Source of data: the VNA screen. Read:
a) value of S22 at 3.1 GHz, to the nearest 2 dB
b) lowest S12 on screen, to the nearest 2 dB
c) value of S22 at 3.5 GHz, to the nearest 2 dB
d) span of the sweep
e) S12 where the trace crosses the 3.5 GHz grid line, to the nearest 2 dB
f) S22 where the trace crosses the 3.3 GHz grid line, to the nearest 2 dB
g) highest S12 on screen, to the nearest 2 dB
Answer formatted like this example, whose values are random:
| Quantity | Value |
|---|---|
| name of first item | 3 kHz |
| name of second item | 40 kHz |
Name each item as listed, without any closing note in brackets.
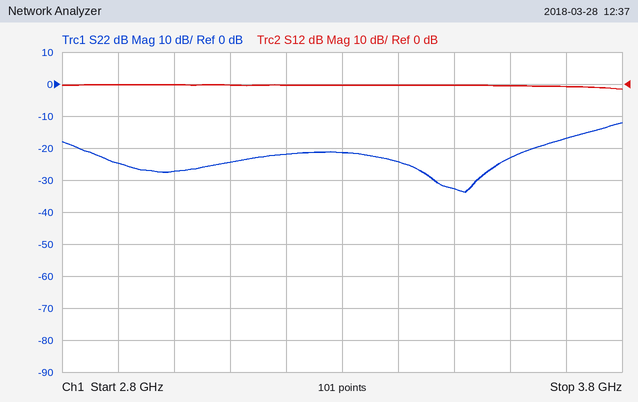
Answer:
| Quantity | Value |
|---|---|
| value of S22 at 3.1 GHz, to the nearest 2 dB | -24 dB |
| lowest S12 on screen, to the nearest 2 dB | -2 dB |
| value of S22 at 3.5 GHz, to the nearest 2 dB | -32 dB |
| span of the sweep | 1 GHz |
| S12 where the trace crosses the 3.5 GHz grid line, to the nearest 2 dB | 0 dB |
| S22 where the trace crosses the 3.3 GHz grid line, to the nearest 2 dB | -22 dB |
| highest S12 on screen, to the nearest 2 dB | 0 dB |
